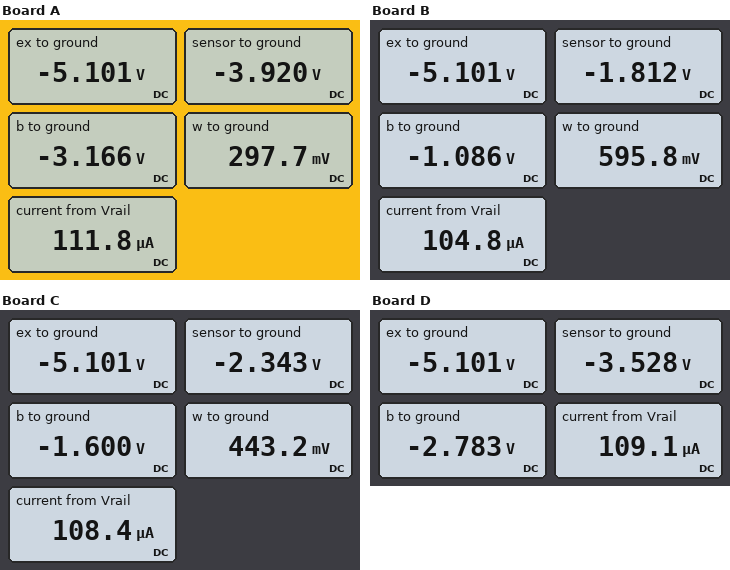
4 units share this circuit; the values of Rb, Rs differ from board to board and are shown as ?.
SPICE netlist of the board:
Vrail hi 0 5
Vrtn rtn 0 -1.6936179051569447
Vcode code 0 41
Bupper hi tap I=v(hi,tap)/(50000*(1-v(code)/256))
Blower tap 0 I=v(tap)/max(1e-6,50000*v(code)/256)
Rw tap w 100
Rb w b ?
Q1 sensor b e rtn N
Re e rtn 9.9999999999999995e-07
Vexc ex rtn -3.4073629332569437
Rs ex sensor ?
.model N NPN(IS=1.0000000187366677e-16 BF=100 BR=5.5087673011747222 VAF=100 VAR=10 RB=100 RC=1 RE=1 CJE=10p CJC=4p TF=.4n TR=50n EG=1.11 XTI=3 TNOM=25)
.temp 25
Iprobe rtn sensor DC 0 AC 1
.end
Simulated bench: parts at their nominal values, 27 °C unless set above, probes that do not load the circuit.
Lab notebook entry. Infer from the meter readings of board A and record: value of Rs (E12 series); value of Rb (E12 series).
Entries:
2.2 kΩ
47 kΩ
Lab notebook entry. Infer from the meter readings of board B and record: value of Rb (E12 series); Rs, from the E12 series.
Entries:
56 kΩ
18 kΩ
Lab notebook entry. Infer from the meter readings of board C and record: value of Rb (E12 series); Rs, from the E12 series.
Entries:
39 kΩ
8.2 kΩ
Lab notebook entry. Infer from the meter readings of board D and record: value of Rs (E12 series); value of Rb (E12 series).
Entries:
3.9 kΩ
56 kΩ
